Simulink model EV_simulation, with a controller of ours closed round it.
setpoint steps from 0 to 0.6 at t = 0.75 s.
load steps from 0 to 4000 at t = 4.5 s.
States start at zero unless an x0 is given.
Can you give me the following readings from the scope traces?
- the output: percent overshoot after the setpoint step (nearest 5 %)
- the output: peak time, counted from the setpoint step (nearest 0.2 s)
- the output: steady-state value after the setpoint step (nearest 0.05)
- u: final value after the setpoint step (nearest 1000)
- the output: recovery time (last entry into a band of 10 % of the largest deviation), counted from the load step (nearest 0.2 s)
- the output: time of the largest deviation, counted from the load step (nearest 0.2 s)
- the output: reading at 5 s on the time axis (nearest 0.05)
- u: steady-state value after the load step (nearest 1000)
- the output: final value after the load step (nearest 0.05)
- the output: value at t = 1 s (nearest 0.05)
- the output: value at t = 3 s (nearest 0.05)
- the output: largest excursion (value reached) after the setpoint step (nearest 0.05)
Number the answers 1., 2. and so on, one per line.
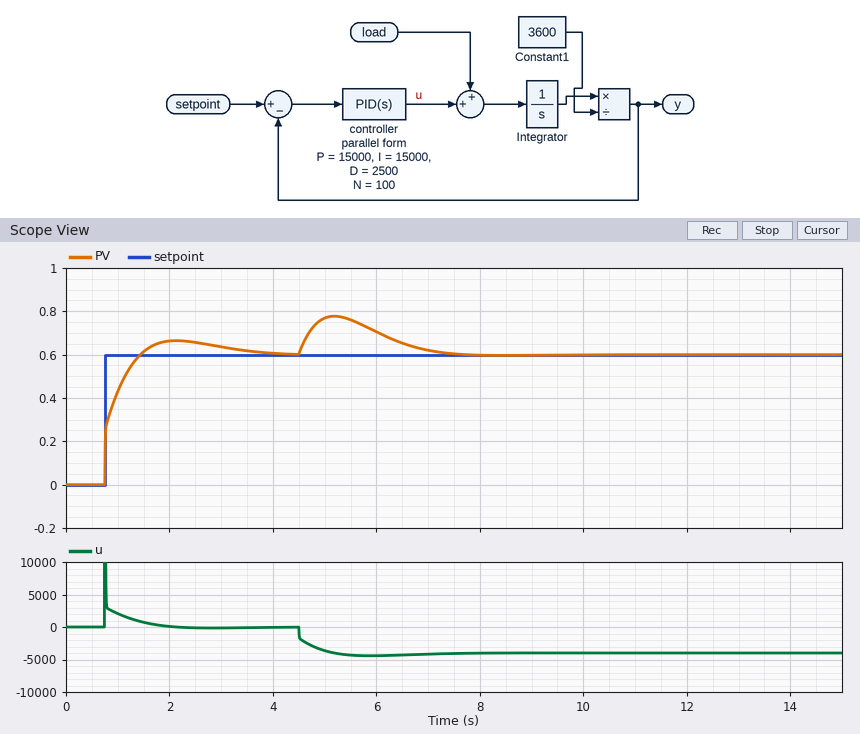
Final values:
1. 10 %
2. 1.4 s
3. 0.60
4. 0
5. 2.6 s
6. 0.6 s
7. 0.75
8. -4000
9. 0.60
10. 0.45
11. 0.65
12. 0.65
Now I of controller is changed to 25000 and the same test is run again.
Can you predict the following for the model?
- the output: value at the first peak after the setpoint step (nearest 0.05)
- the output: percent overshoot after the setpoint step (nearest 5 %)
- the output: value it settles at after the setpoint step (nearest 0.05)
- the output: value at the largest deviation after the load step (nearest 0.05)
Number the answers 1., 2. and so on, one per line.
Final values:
1. 0.70
2. 15 %
3. 0.60
4. 0.75
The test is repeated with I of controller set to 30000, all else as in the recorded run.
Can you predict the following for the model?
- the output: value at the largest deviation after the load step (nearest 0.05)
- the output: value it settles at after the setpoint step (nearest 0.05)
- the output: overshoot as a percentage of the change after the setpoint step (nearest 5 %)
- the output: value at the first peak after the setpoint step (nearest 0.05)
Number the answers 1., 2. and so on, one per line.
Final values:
1. 0.75
2. 0.60
3. 15 %
4. 0.70
